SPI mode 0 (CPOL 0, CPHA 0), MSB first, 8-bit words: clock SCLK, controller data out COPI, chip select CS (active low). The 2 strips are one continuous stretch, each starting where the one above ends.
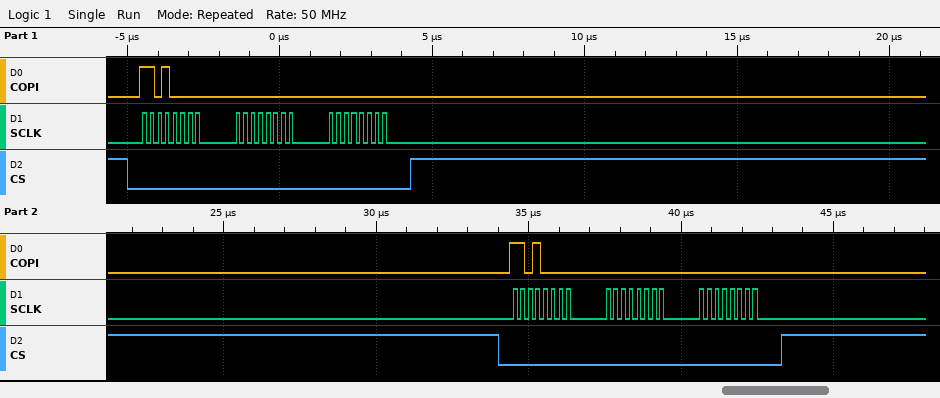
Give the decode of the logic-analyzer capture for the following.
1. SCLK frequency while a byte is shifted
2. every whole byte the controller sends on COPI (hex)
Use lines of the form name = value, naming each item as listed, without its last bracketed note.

SCLK frequency while a byte is shifted = 4 MHz
every whole byte the controller sends on COPI = D0 00 00 D0 00 00
